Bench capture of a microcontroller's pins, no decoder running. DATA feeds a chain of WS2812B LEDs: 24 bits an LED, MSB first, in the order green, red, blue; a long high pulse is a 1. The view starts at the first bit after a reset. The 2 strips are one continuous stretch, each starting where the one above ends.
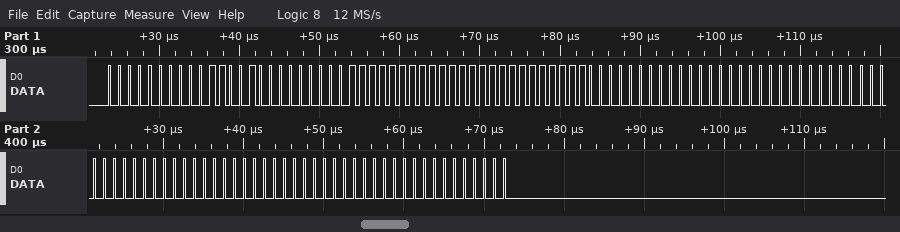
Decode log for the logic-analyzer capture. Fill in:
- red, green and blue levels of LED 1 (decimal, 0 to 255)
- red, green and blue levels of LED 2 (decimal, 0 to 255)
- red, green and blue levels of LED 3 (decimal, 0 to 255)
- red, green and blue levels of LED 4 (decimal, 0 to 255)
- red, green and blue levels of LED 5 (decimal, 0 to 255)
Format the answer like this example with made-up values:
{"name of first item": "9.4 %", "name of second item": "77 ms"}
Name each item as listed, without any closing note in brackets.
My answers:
{"red, green and blue levels of LED 1": "50, 0, 0", "red, green and blue levels of LED 2": "255, 255, 255", "red, green and blue levels of LED 3": "0, 0, 0", "red, green and blue levels of LED 4": "0, 0, 0", "red, green and blue levels of LED 5": "0, 0, 0"}
